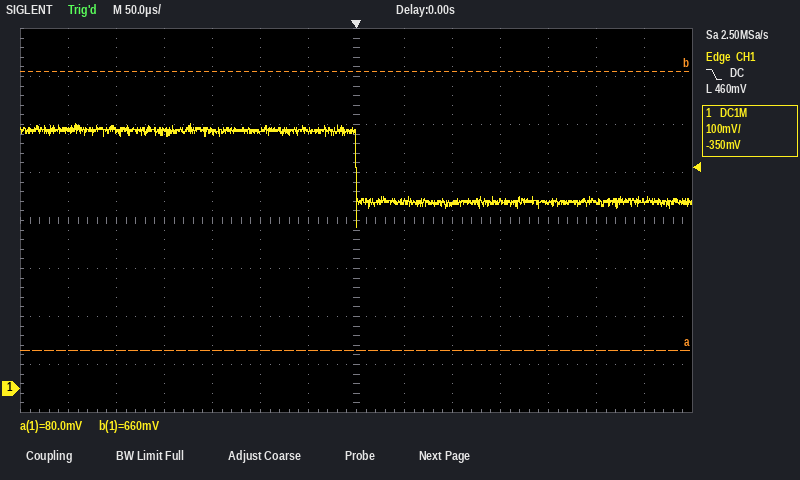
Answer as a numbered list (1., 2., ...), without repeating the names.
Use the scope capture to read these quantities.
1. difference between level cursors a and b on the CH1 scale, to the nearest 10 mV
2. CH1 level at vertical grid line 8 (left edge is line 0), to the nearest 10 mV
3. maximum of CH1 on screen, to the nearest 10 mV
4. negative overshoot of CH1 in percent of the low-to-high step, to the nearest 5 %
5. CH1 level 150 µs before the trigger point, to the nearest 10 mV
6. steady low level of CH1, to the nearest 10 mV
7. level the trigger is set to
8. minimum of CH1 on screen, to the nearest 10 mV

1. 580 mV
2. 390 mV
3. 550 mV
4. 35 %
5. 540 mV
6. 390 mV
7. 460 mV
8. 340 mV
